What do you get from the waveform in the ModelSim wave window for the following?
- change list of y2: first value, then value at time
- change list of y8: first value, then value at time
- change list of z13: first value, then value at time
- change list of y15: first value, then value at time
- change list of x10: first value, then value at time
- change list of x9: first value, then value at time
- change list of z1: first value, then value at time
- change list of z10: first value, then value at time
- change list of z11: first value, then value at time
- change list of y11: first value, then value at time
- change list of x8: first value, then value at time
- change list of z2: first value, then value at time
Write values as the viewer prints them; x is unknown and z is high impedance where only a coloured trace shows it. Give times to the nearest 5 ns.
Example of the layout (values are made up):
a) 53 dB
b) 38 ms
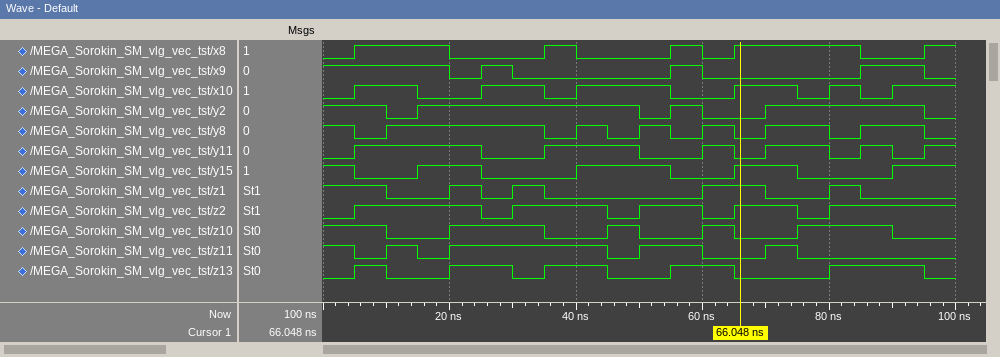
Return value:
a) 1, 0 at 10 ns, 1 at 15 ns, 0 at 50 ns, 1 at 55 ns, 0 at 60 ns, 1 at 70 ns, 0 at 95 ns
b) 1, 0 at 5 ns, 1 at 10 ns, 0 at 35 ns, 1 at 40 ns, 0 at 45 ns, 1 at 50 ns, 0 at 55 ns, 1 at 60 ns, 0 at 65 ns, 1 at 70 ns, 0 at 80 ns, 1 at 85 ns, 0 at 95 ns
c) 0, 1 at 5 ns, 0 at 10 ns, 1 at 20 ns, 0 at 30 ns, 1 at 35 ns, 0 at 45 ns, 1 at 55 ns, 0 at 65 ns, 1 at 80 ns, 0 at 95 ns
d) 1, 0 at 5 ns, 1 at 15 ns, 0 at 25 ns, 1 at 40 ns, 0 at 55 ns, 1 at 65 ns, 0 at 75 ns, 1 at 90 ns
e) 0, 1 at 5 ns, 0 at 15 ns, 1 at 25 ns, 0 at 35 ns, 1 at 40 ns, 0 at 55 ns, 1 at 65 ns, 0 at 75 ns, 1 at 80 ns, 0 at 85 ns, 1 at 90 ns
f) 1, 0 at 20 ns, 1 at 25 ns, 0 at 30 ns, 1 at 55 ns, 0 at 60 ns, 1 at 85 ns, 0 at 95 ns
g) 1, 0 at 10 ns, 1 at 20 ns, 0 at 25 ns, 1 at 30 ns, 0 at 35 ns, 1 at 60 ns, 0 at 70 ns, 1 at 80 ns, 0 at 85 ns
h) 1, 0 at 10 ns, 1 at 20 ns, 0 at 35 ns, 1 at 45 ns, 0 at 50 ns, 1 at 60 ns, 0 at 65 ns, 1 at 75 ns, 0 at 90 ns
i) 1, 0 at 5 ns, 1 at 10 ns, 0 at 15 ns, 1 at 20 ns, 0 at 45 ns, 1 at 50 ns, 0 at 60 ns, 1 at 70 ns, 0 at 75 ns
j) 0, 1 at 5 ns, 0 at 25 ns, 1 at 35 ns, 0 at 50 ns, 1 at 60 ns, 0 at 65 ns, 1 at 70 ns, 0 at 80 ns, 1 at 85 ns, 0 at 90 ns, 1 at 95 ns
k) 0, 1 at 5 ns, 0 at 20 ns, 1 at 35 ns, 0 at 40 ns, 1 at 55 ns, 0 at 60 ns, 1 at 65 ns, 0 at 85 ns, 1 at 95 ns
l) 0, 1 at 5 ns, 0 at 25 ns, 1 at 30 ns, 0 at 45 ns, 1 at 50 ns, 0 at 60 ns, 1 at 65 ns, 0 at 75 ns, 1 at 80 ns
